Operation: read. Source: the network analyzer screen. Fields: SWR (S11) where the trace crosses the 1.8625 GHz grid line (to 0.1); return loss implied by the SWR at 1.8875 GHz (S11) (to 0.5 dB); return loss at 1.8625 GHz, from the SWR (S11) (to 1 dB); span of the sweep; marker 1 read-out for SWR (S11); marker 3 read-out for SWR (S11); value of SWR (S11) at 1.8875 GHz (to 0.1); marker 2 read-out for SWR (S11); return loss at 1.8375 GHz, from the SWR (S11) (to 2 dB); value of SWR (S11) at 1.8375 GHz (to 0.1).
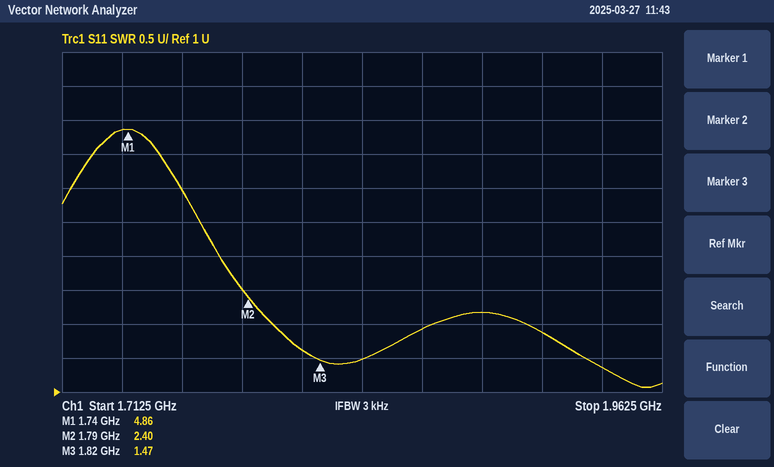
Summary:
1.9
8.5 dB
10 dB
250 MHz
4.86
1.47
2.2
2.40
14 dB
1.5
